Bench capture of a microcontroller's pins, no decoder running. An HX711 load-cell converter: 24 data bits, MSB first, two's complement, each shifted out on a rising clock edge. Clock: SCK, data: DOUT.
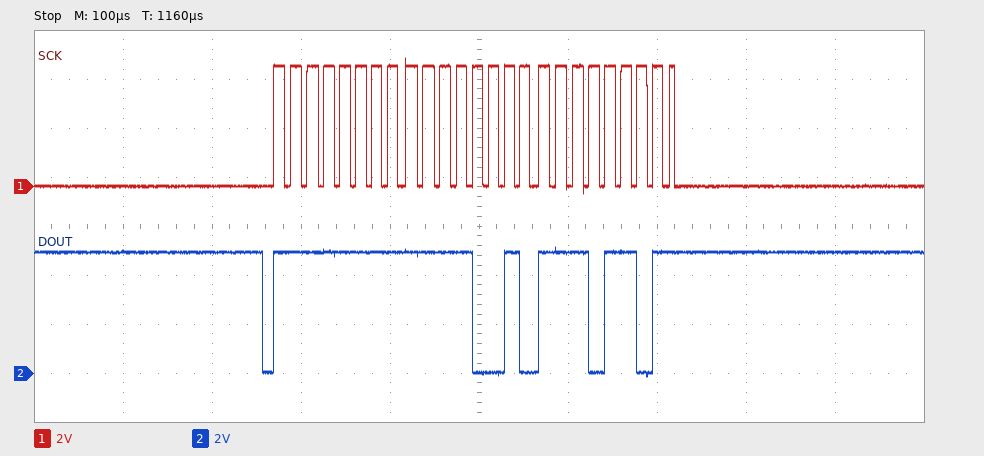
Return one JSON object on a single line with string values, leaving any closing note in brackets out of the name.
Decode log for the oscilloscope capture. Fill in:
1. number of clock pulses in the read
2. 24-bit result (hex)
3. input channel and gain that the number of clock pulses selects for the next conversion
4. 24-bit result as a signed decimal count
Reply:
{"number of clock pulses in the read": "25", "24-bit result": "0xFFF2ED", "input channel and gain that the number of clock pulses selects for the next conversion": "channel A, gain 128", "24-bit result as a signed decimal count": "-3347"}
